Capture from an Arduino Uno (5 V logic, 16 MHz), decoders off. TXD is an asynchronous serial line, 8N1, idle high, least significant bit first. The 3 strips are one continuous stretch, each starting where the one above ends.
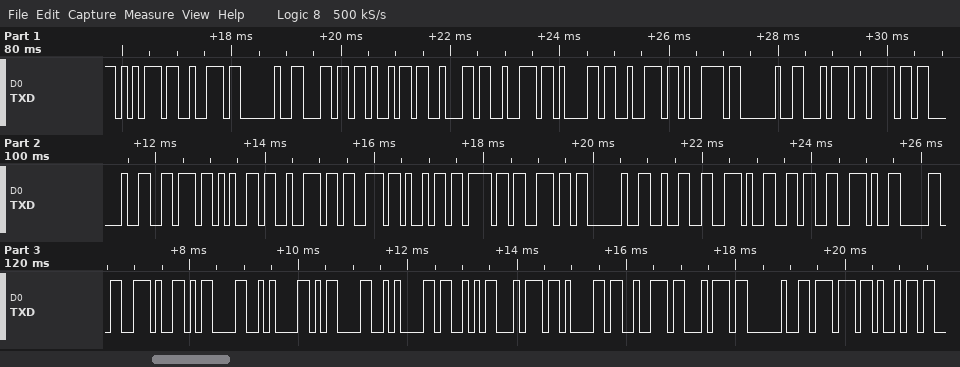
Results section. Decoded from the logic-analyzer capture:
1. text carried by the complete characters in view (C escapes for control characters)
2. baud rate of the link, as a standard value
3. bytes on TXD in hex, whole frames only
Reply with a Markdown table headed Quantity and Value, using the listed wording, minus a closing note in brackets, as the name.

| Quantity | Value |
|---|---|
| text carried by the complete characters in view | "ur library to version 2.6.0.\r\n\r\nStart wi" |
| baud rate of the link, as a standard value | 9600 baud |
| bytes on TXD in hex, whole frames only | 75 72 20 6C 69 62 72 61 72 79 20 74 6F 20 76 65 72 73 69 6F 6E 20 32 2E 36 2E 30 2E 0D 0A 0D 0A 53 74 61 72 74 20 77 69 |
